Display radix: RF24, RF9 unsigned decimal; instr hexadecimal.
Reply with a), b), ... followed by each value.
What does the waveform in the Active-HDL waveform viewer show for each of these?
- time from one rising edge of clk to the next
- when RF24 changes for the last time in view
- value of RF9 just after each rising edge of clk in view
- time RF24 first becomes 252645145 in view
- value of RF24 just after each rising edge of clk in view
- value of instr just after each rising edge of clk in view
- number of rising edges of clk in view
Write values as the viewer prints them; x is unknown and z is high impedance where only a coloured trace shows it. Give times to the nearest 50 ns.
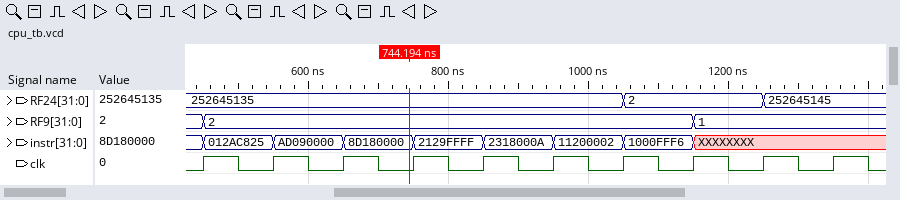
a) 100 ns
b) 1250 ns
c) 2, 2, 2, 2, 2, 2, 2, 1, 1, 1
d) 1250 ns
e) 252645135, 252645135, 252645135, 252645135, 252645135, 252645135, 2, 2, 252645145, 252645145
f) 012AC825, AD090000, 8D180000, 2129FFFF, 2318000A, 11200002, 1000FFF6, XXXXXXXX, XXXXXXXX, XXXXXXXX
g) 10
